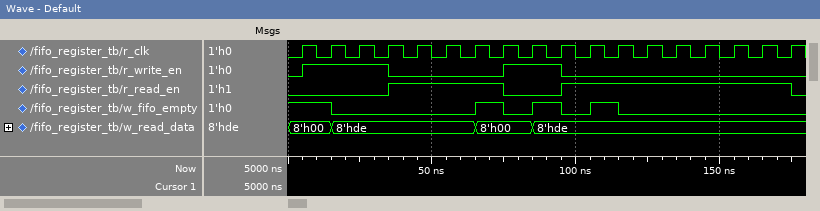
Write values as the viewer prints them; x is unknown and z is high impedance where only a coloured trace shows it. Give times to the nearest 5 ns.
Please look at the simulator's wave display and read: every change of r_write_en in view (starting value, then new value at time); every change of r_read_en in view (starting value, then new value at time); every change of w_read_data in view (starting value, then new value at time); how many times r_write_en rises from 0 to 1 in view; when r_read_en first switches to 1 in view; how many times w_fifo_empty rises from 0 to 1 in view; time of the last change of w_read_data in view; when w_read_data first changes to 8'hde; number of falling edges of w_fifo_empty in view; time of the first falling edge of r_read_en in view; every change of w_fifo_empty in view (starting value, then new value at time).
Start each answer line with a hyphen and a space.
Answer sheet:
- 0, 1 at 5 ns, 0 at 35 ns, 1 at 75 ns, 0 at 95 ns
- 0, 1 at 35 ns, 0 at 75 ns, 1 at 95 ns, 0 at 175 ns
- 8'h00, 8'hde at 15 ns, 8'h00 at 65 ns, 8'hde at 85 ns
- 2
- 35 ns
- 3
- 85 ns
- 15 ns
- 4
- 75 ns
- 1, 0 at 15 ns, 1 at 65 ns, 0 at 75 ns, 1 at 85 ns, 0 at 95 ns, 1 at 105 ns, 0 at 115 ns
